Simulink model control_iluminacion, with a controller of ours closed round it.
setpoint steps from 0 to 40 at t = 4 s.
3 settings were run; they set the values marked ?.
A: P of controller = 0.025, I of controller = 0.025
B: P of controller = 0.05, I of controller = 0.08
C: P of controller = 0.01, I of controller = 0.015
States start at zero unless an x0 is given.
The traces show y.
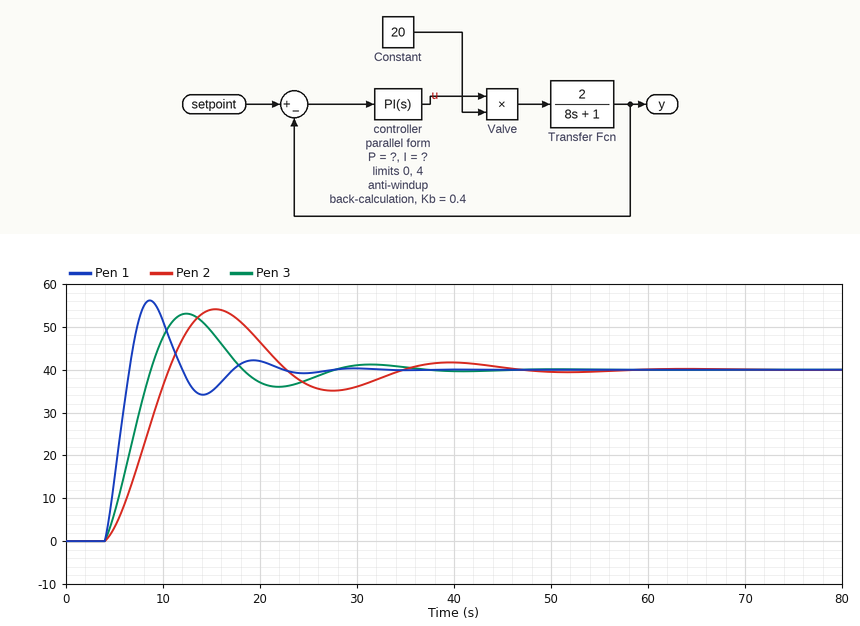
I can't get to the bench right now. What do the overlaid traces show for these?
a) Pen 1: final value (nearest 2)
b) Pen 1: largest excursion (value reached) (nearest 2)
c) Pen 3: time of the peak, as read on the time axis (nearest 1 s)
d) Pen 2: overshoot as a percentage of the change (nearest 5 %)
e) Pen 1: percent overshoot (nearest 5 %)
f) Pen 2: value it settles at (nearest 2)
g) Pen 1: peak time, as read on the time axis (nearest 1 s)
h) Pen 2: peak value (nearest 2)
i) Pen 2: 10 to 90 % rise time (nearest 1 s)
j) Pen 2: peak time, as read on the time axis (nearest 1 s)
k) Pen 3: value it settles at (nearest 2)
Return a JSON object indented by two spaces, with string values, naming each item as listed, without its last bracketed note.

{
  "Pen 1: final value": "40",
  "Pen 1: largest excursion (value reached)": "56",
  "Pen 3: time of the peak, as read on the time axis": "12 s",
  "Pen 2: overshoot as a percentage of the change": "35 %",
  "Pen 1: percent overshoot": "40 %",
  "Pen 2: value it settles at": "40",
  "Pen 1: peak time, as read on the time axis": "9 s",
  "Pen 2: peak value": "54",
  "Pen 2: 10 to 90 % rise time": "5 s",
  "Pen 2: peak time, as read on the time axis": "15 s",
  "Pen 3: value it settles at": "40"
}
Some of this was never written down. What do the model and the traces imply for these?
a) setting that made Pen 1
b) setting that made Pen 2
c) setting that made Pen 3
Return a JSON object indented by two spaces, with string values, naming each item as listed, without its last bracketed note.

{
  "setting that made Pen 1": "B",
  "setting that made Pen 2": "C",
  "setting that made Pen 3": "A"
}
